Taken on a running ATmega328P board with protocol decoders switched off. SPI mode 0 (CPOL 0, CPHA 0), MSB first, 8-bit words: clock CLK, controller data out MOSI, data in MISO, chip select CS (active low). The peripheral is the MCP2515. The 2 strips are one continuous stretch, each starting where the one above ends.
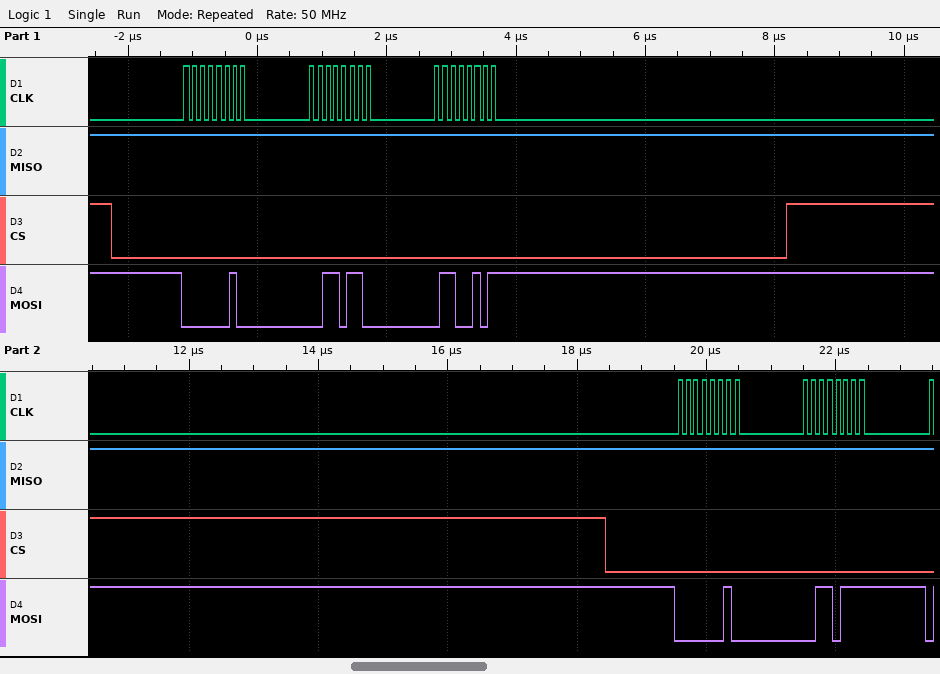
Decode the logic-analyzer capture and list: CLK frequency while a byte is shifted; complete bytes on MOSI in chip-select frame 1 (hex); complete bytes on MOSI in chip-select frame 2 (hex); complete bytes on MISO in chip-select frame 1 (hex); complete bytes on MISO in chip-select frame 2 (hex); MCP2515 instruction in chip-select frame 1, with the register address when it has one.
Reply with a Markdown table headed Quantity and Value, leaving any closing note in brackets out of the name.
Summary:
| Quantity | Value |
|---|---|
| CLK frequency while a byte is shifted | 8 MHz |
| complete bytes on MOSI in chip-select frame 1 | 0x02 0x36 0x65 |
| complete bytes on MOSI in chip-select frame 2 | 0x02 0x37 |
| complete bytes on MISO in chip-select frame 1 | 0xFF 0xFF 0xFF |
| complete bytes on MISO in chip-select frame 2 | 0xFF 0xFF |
| MCP2515 instruction in chip-select frame 1, with the register address when it has one | WRITE 0x36 |
